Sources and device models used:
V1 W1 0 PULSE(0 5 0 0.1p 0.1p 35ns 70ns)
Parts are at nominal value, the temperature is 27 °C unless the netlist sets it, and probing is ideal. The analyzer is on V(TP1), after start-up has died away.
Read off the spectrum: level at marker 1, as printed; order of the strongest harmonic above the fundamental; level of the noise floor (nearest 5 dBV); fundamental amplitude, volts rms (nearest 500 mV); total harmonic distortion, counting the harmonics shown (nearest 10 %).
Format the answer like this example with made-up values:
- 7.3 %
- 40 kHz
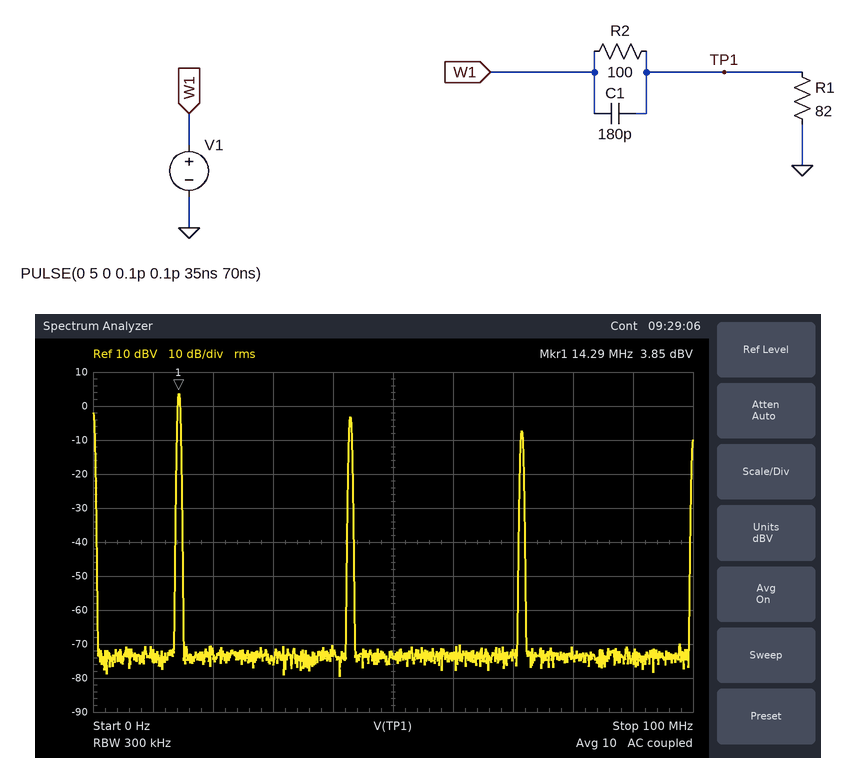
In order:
- 3.85 dBV
- 3
- -75 dBV
- 1.5 V
- 50 %
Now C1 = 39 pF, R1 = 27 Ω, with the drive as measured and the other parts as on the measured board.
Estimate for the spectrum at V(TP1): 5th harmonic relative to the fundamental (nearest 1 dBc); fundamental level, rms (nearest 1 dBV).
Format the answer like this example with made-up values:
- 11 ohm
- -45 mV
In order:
- -9 dBc
- -6 dBV
